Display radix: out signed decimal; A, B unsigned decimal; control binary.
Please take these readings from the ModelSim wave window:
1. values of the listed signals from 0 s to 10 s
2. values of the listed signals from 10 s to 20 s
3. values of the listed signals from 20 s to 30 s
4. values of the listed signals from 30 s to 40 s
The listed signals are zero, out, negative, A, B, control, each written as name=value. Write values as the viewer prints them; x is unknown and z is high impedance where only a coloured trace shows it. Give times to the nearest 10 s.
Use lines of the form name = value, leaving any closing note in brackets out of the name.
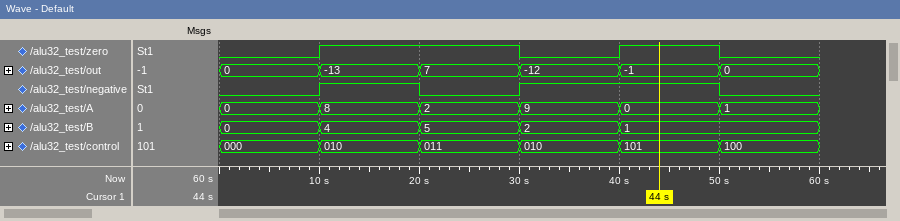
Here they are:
values of the listed signals from 0 s to 10 s = zero=0, out=0, negative=0, A=0, B=0, control=000
values of the listed signals from 10 s to 20 s = zero=1, out=-13, negative=1, A=8, B=4, control=010
values of the listed signals from 20 s to 30 s = zero=1, out=7, negative=0, A=2, B=5, control=011
values of the listed signals from 30 s to 40 s = zero=0, out=-12, negative=1, A=9, B=2, control=010
